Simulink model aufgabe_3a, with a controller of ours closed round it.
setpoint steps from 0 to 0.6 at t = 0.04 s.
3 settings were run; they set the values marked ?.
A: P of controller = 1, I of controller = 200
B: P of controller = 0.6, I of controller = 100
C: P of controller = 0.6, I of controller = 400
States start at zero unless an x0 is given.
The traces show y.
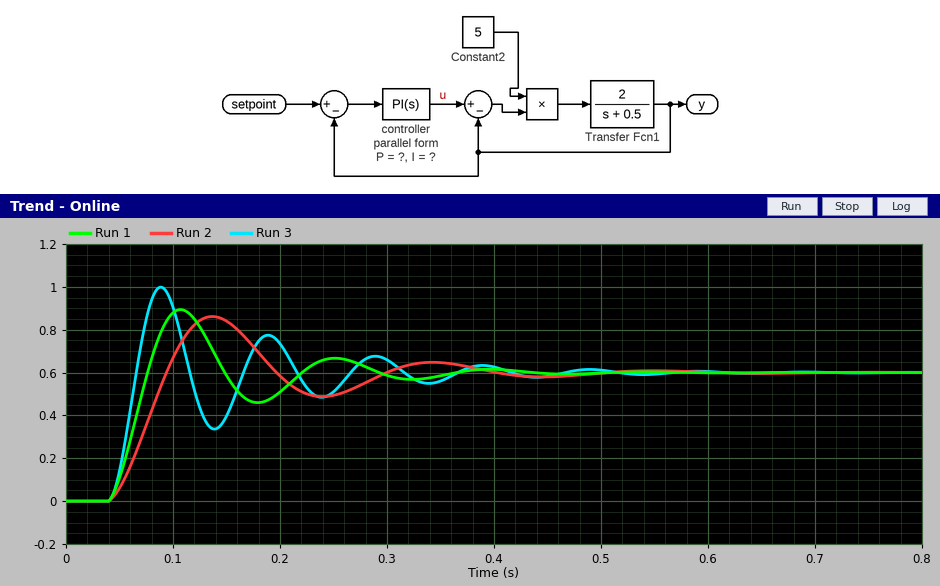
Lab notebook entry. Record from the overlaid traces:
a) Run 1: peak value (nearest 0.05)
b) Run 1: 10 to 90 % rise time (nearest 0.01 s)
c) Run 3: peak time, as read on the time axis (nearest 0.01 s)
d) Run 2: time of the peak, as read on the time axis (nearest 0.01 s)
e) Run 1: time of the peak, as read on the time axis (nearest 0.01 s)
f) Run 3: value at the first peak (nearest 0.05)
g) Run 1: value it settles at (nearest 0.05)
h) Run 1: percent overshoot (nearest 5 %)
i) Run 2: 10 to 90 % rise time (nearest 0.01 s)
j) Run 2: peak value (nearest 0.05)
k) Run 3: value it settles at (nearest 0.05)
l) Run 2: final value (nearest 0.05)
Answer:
0.90
0.03 s
0.09 s
0.14 s
0.11 s
1.00
0.60
50 %
0.04 s
0.85
0.60
0.60
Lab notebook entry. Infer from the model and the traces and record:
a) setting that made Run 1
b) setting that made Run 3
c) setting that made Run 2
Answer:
A
C
B
